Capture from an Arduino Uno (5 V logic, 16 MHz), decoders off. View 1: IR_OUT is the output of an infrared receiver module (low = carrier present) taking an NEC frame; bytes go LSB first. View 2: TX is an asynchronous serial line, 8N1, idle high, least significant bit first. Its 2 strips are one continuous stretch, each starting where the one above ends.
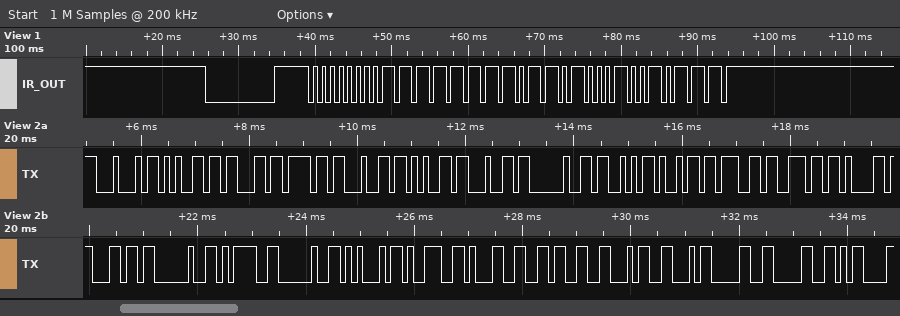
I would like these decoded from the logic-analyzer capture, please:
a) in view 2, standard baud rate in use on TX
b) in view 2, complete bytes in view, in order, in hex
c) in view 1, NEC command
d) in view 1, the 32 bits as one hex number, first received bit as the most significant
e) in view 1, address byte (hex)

9600 baud
44 65 63 6F 64 65 64 20 53 69 67 6E 61 6C 20 3D 20 45 39 31 36 46 46 30 30 0D
0x16
0x00FF6897
0x00
